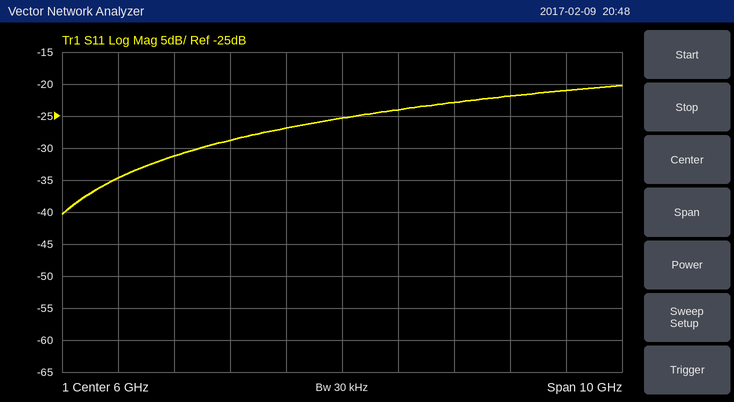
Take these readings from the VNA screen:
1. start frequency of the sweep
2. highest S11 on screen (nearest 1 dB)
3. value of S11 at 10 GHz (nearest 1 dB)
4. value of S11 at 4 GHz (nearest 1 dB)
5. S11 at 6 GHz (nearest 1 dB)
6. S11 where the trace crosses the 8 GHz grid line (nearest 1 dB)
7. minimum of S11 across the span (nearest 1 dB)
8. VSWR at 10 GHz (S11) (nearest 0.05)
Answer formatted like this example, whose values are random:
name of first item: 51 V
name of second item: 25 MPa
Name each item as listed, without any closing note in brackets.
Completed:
start frequency of the sweep: 1 GHz
highest S11 on screen: -20 dB
value of S11 at 10 GHz: -21 dB
value of S11 at 4 GHz: -29 dB
S11 at 6 GHz: -25 dB
S11 where the trace crosses the 8 GHz grid line: -23 dB
minimum of S11 across the span: -40 dB
VSWR at 10 GHz (S11): 1.20
